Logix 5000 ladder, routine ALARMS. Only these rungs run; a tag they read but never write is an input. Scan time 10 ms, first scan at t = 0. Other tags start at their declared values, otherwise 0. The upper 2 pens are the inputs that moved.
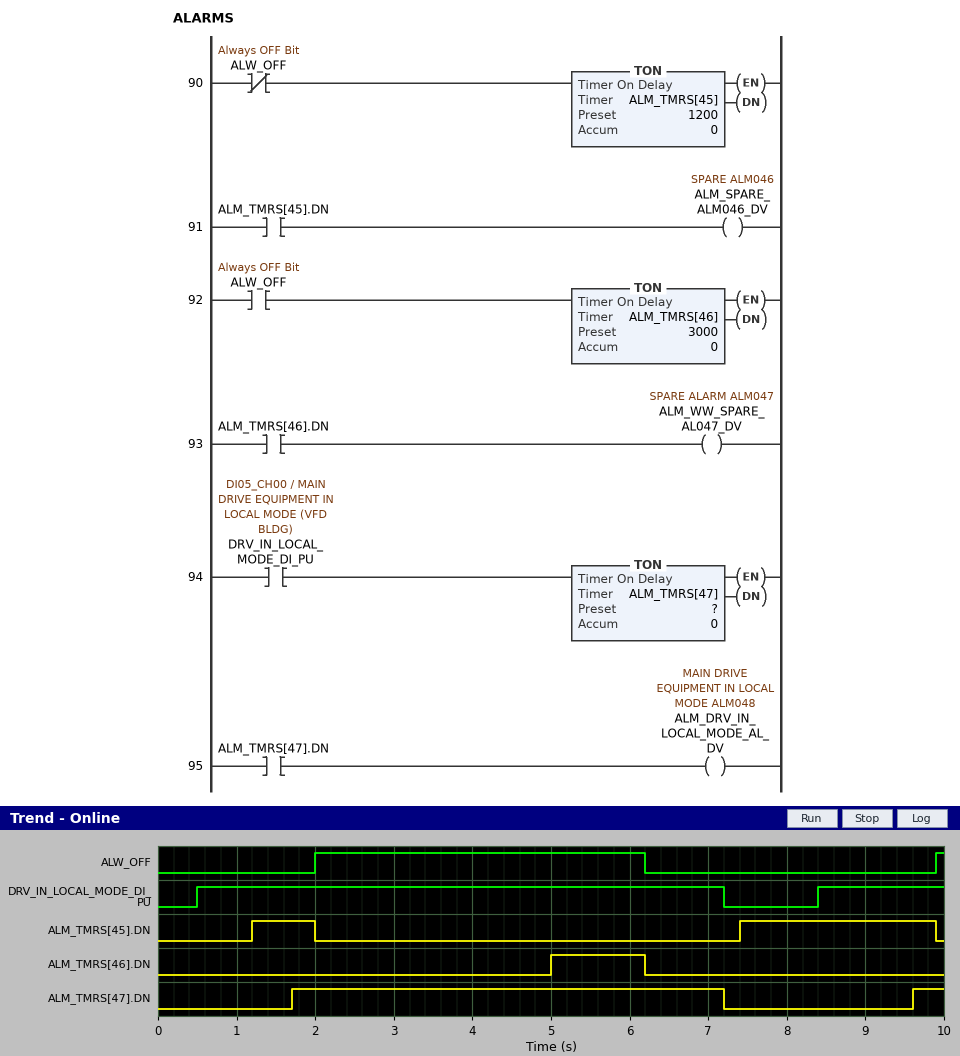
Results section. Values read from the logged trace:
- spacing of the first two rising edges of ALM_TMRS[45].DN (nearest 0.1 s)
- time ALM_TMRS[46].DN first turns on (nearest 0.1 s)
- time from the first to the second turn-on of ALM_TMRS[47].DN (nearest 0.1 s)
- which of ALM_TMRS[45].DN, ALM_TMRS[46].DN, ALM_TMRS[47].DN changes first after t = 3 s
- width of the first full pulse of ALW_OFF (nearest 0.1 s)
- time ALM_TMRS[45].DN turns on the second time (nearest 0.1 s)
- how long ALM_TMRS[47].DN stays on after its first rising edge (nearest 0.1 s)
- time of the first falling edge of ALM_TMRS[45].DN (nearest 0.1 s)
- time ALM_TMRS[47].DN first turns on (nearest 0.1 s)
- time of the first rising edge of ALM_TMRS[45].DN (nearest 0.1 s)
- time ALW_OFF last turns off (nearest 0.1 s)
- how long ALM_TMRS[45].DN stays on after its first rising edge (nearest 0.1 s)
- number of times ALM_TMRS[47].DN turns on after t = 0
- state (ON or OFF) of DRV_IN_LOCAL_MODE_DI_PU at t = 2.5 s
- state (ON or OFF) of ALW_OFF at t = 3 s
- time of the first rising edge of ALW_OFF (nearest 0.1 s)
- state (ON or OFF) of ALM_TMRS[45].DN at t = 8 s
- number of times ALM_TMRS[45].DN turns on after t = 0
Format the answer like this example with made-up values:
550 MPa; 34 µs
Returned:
6.2 s; 5.0 s; 7.9 s; ALM_TMRS[46].DN; 4.2 s; 7.4 s; 5.5 s; 2.0 s; 1.7 s; 1.2 s; 6.2 s; 0.8 s; 2; ON; ON; 2.0 s; ON; 2
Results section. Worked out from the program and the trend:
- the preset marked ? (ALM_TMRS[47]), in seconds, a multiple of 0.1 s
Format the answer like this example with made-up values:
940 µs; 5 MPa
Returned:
1.2 s
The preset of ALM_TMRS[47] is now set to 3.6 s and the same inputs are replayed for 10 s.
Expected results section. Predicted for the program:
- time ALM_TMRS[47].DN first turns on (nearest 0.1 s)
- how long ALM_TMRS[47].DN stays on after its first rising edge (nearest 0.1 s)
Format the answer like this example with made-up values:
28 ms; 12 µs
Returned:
4.1 s; 3.1 s
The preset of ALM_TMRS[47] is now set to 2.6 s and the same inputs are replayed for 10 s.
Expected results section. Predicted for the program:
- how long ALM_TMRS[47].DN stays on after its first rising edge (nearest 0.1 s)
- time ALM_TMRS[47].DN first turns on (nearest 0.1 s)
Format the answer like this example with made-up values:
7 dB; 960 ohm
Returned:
4.1 s; 3.1 s
